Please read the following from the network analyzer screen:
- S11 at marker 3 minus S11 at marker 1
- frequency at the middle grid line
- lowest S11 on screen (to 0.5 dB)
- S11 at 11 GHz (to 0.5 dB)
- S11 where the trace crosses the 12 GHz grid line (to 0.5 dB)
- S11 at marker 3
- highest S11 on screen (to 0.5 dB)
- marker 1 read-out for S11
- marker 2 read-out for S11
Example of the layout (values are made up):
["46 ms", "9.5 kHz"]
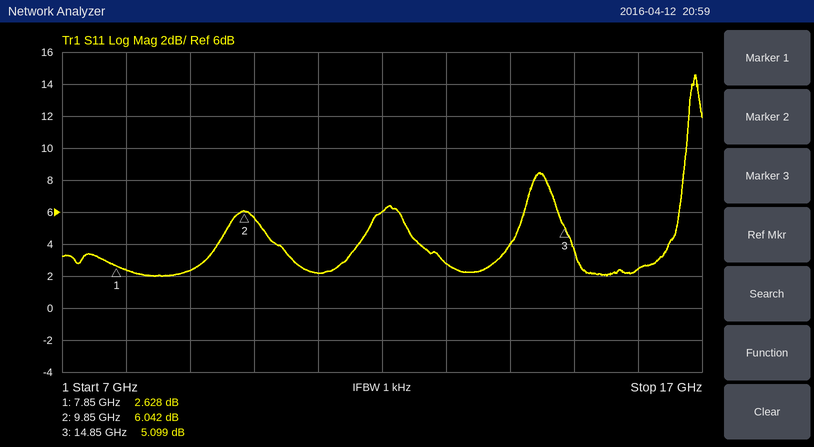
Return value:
["2.471 dB", "12 GHz", "2.0 dB", "2.0 dB", "6.0 dB", "5.099 dB", "14.5 dB", "2.628 dB", "6.042 dB"]
